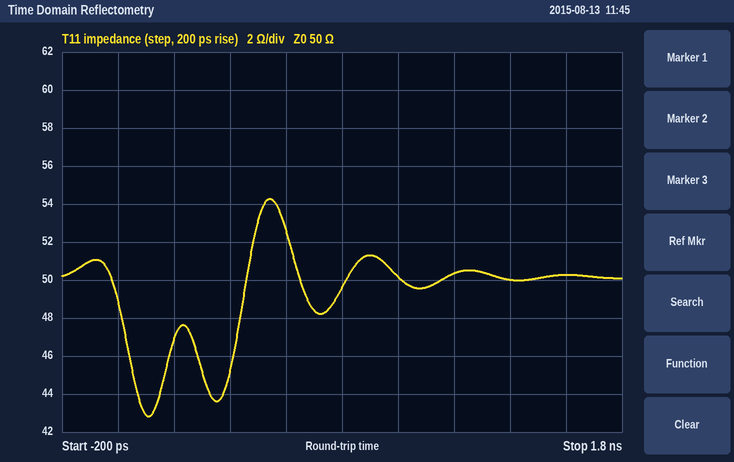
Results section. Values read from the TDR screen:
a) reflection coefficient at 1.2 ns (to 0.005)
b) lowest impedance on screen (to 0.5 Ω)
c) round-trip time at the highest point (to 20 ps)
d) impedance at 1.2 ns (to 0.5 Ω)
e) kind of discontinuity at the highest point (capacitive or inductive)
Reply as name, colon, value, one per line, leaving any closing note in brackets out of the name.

reflection coefficient at 1.2 ns: +0.005
lowest impedance on screen: 43.0 Ω
round-trip time at the highest point: 540 ps
impedance at 1.2 ns: 50.5 Ω
kind of discontinuity at the highest point: inductive
